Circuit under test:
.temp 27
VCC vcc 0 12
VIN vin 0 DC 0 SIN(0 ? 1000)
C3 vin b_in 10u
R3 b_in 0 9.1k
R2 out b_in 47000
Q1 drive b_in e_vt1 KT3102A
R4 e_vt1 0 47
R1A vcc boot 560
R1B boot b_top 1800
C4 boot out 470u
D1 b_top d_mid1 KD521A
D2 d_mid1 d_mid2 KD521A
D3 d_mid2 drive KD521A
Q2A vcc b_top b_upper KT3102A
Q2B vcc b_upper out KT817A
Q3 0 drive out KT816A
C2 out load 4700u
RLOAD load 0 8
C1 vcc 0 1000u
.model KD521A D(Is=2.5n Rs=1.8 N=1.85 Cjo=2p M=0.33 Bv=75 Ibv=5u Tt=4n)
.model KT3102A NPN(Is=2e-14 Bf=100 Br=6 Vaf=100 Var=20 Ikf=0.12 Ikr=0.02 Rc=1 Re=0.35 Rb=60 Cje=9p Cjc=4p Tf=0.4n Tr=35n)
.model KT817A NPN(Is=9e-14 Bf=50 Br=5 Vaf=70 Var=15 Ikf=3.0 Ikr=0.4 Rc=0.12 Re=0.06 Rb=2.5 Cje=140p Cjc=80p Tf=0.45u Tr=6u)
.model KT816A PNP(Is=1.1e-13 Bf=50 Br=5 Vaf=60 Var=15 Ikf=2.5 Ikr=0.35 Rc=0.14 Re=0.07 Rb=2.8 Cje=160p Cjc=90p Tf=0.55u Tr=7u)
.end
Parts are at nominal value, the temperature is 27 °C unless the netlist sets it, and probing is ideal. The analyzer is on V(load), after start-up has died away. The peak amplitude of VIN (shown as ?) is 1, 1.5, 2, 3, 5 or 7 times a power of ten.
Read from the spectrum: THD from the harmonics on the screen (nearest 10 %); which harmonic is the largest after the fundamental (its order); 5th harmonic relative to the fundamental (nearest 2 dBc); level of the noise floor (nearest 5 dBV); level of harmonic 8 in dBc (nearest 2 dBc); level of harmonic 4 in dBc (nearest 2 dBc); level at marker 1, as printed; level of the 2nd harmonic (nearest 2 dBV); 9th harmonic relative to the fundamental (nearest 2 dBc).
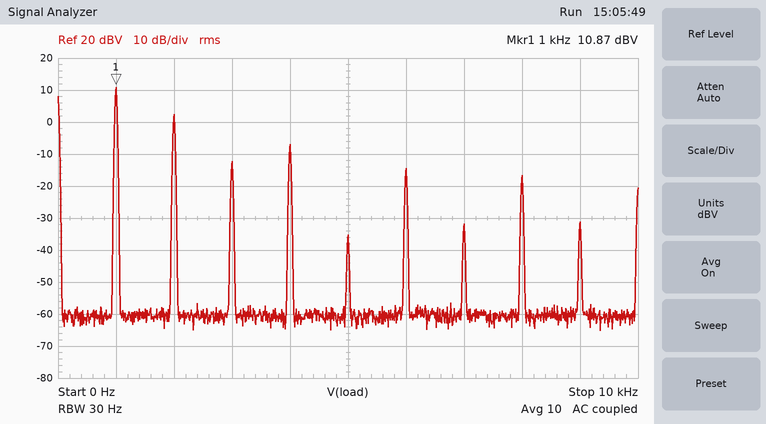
40 %
2
-46 dBc
-60 dBV
-28 dBc
-18 dBc
10.87 dBV
2 dBV
-42 dBc
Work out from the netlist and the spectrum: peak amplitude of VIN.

1.5 V
